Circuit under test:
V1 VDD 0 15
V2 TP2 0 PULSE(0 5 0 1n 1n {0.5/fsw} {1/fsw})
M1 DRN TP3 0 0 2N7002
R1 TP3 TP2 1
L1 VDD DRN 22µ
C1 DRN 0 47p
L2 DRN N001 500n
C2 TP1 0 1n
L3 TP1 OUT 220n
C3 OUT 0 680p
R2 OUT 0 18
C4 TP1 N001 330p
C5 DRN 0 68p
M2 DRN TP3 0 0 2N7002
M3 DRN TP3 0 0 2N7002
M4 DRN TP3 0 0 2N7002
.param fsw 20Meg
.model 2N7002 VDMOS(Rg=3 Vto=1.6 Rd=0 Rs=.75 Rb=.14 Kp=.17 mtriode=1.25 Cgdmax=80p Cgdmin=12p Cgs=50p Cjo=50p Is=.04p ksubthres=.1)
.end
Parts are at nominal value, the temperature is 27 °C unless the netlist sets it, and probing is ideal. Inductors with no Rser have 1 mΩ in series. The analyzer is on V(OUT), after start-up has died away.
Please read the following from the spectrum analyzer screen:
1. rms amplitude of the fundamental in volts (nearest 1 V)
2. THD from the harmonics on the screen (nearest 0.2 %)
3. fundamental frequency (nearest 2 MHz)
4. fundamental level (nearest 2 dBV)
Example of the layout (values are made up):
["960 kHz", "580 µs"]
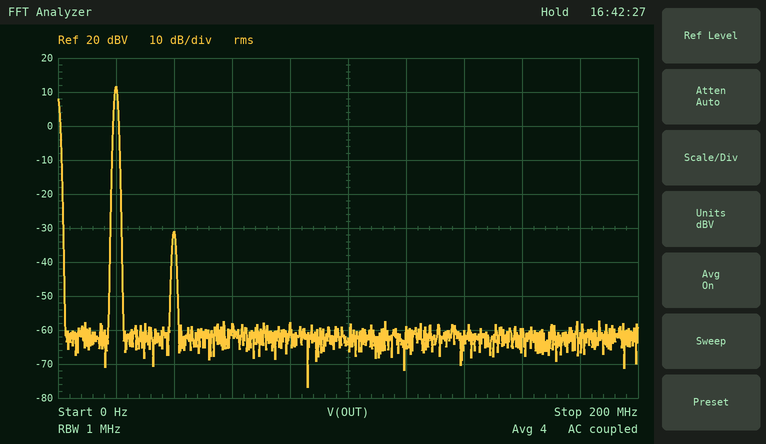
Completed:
["4 V", "0.8 %", "20 MHz", "12 dBV"]
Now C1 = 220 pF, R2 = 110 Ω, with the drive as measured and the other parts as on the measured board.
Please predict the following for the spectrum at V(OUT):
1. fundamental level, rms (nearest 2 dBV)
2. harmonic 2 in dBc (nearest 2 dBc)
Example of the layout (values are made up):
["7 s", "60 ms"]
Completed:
["18 dBV", "-50 dBc"]
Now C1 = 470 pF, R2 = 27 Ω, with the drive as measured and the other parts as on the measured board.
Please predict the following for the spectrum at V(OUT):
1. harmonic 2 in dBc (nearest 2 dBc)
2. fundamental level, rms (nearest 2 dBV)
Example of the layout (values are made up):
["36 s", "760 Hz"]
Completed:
["-50 dBc", "12 dBV"]
